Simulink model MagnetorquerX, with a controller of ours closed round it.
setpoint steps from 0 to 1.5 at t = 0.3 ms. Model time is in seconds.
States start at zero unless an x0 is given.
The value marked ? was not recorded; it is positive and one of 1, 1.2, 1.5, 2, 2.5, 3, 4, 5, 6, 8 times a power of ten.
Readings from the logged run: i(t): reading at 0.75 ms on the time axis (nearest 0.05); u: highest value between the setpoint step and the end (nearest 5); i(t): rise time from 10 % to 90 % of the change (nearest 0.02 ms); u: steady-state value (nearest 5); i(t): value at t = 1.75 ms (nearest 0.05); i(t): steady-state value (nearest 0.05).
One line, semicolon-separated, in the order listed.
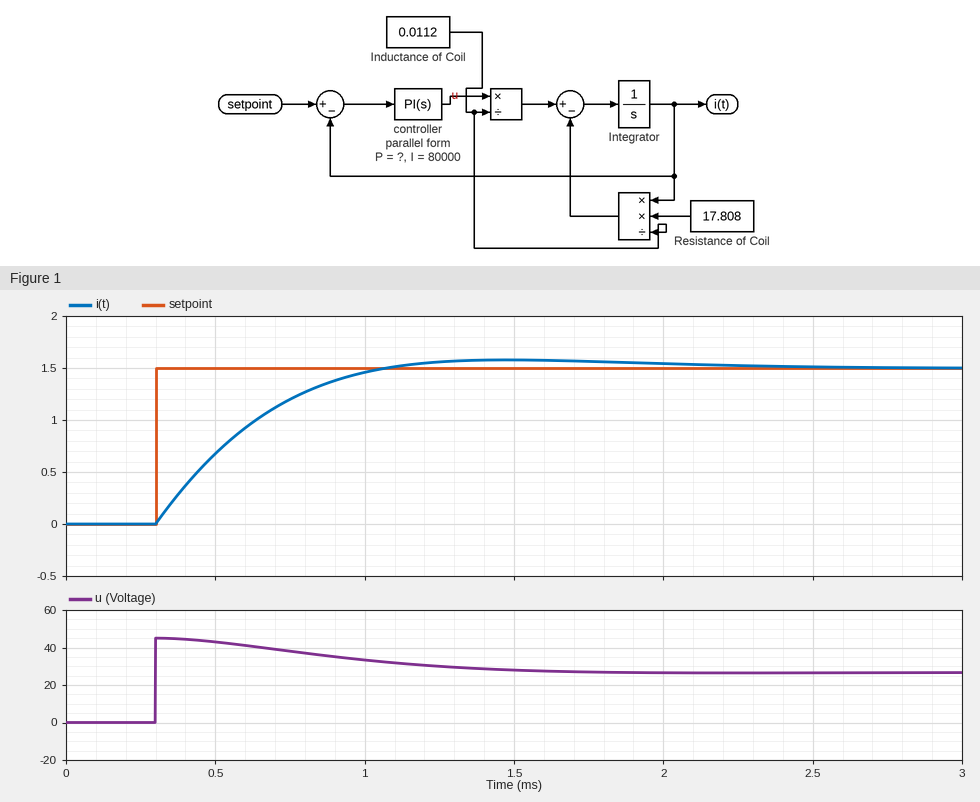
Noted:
1.20; 45; 0.54 ms; 25; 1.55; 1.50
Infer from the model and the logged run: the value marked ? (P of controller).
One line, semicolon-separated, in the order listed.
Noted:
30
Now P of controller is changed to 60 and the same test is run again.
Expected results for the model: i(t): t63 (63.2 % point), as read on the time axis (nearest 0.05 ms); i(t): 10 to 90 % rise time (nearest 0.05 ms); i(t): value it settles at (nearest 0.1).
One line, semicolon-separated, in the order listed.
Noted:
0.50 ms; 0.45 ms; 1.5
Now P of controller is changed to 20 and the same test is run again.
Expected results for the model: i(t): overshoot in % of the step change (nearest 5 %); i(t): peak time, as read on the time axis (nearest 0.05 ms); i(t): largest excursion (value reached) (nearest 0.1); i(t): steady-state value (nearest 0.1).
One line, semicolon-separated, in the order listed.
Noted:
10 %; 1.45 ms; 1.7; 1.5
